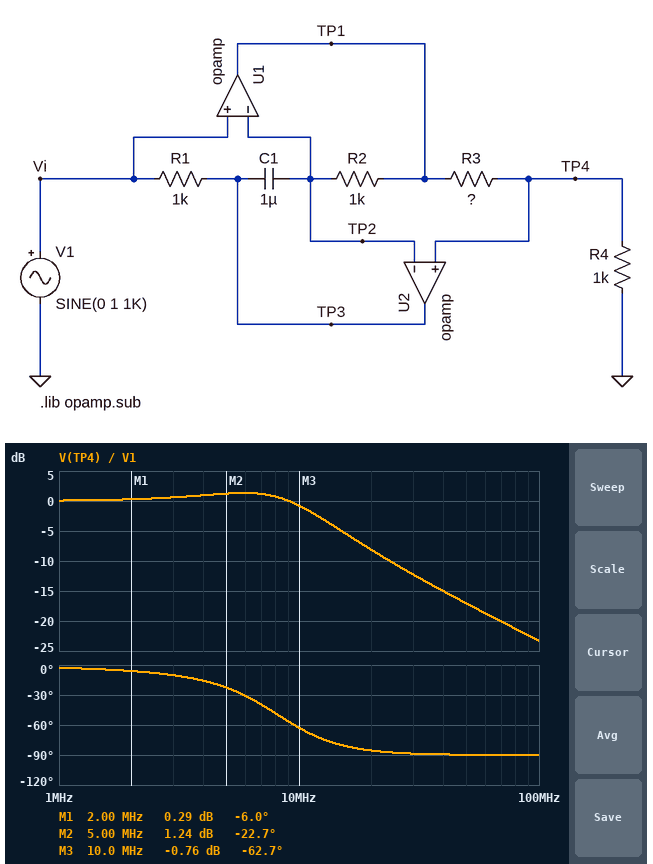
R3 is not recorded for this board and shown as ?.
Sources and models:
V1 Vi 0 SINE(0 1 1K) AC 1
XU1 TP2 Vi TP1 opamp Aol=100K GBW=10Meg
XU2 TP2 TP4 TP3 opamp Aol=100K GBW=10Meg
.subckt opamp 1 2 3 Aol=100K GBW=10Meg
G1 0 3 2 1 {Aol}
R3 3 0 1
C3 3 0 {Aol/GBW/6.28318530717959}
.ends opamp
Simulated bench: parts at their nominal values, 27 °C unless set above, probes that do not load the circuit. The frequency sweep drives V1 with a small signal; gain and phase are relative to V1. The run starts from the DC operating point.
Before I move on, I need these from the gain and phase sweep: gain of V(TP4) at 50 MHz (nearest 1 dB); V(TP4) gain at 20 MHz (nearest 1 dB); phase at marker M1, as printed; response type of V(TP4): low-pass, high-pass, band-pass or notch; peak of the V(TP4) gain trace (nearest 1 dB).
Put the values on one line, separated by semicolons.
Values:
-17 dB; -8 dB; -6.0 deg; low-pass; 1 dB
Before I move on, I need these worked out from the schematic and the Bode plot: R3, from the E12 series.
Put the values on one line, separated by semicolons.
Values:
470 Ω
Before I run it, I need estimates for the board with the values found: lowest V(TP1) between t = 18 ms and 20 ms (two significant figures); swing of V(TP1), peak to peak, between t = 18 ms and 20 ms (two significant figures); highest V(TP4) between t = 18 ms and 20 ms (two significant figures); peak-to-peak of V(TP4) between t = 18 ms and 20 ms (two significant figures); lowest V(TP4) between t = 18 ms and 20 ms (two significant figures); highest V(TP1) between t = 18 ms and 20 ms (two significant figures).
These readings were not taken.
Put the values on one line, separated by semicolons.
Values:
-1.5 V; 2.9 V; 1.0 V; 2.0 V; -1.0 V; 1.5 V
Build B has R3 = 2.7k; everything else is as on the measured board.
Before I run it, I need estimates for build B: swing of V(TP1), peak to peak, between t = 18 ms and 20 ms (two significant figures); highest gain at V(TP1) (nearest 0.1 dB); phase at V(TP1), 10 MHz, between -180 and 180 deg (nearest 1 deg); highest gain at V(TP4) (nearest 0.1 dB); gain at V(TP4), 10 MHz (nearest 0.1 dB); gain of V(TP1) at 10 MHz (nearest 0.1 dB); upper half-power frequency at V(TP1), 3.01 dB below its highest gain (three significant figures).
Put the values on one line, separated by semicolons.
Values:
7.4 V; 11.4 dB; -81 deg; 0 dB; -10.2 dB; 1.2 dB; 3.95 MHz
